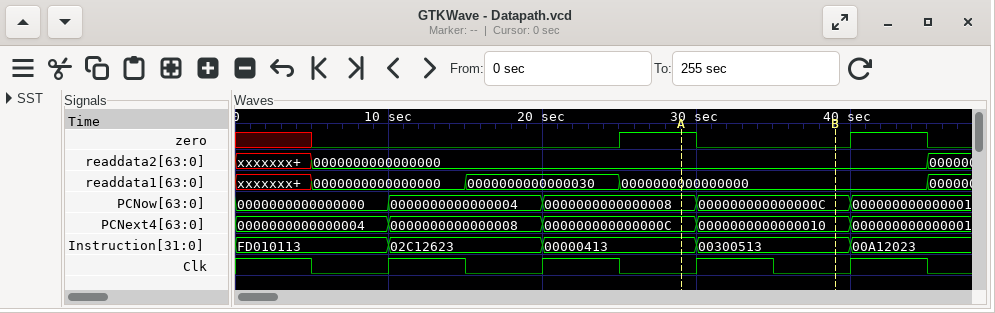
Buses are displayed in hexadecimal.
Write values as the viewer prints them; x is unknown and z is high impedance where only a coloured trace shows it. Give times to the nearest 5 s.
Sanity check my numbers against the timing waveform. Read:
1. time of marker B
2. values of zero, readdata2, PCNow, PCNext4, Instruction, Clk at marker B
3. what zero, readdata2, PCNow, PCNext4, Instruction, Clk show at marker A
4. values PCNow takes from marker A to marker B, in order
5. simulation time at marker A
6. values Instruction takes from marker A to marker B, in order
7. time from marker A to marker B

40 s
zero=0, readdata2=0000000000000000, PCNow=000000000000000C, PCNext4=0000000000000010, Instruction=00300513, Clk=0
zero=1, readdata2=0000000000000000, PCNow=0000000000000008, PCNext4=000000000000000C, Instruction=00000413, Clk=0
0000000000000008, 000000000000000C
30 s
00000413, 00300513
10 s
